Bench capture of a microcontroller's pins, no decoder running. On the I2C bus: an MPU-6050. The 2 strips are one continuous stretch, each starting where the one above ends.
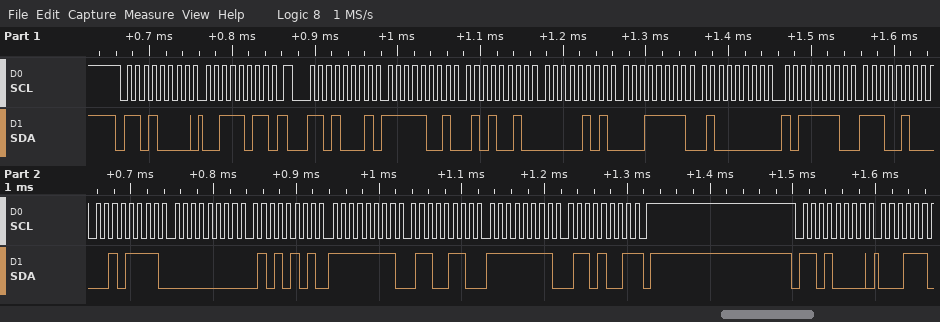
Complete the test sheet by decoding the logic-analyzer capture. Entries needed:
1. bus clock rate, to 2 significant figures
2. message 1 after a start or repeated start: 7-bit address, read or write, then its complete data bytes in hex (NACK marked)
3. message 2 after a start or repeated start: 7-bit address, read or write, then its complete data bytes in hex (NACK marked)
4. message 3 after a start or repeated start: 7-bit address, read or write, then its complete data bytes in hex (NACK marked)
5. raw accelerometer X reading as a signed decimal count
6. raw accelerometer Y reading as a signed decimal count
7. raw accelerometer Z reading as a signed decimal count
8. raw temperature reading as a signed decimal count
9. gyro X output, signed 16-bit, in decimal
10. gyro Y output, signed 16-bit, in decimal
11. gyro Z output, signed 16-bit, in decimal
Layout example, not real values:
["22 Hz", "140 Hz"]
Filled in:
["100 kHz", "0x68 write: 3B", "0x68 read: F9 52 05 1F 40 BE E4 2F 00 55 FF 66 FF 69 NACK", "0x68 write", "-1710", "1311", "16574", "-7121", "85", "-154", "-151"]
